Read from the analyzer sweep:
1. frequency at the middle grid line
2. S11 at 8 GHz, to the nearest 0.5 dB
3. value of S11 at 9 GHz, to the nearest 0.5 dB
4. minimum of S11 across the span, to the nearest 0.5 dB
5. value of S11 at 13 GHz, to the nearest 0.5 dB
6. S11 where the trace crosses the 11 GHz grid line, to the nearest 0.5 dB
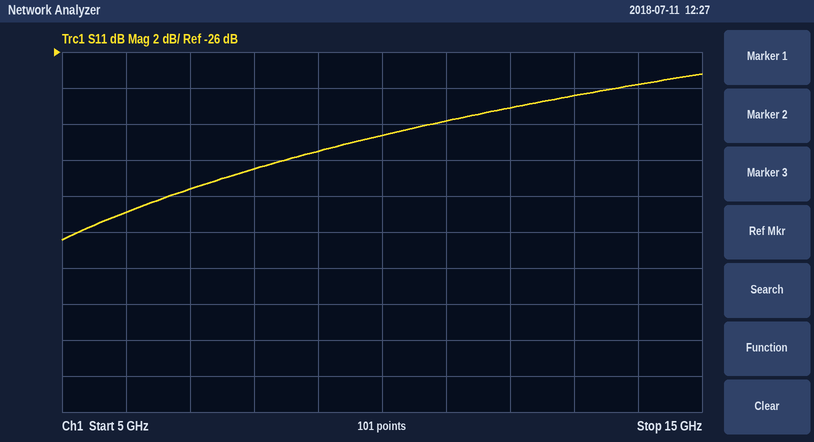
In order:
10 GHz
-32.5 dB
-31.5 dB
-36.5 dB
-28.5 dB
-30.0 dB
